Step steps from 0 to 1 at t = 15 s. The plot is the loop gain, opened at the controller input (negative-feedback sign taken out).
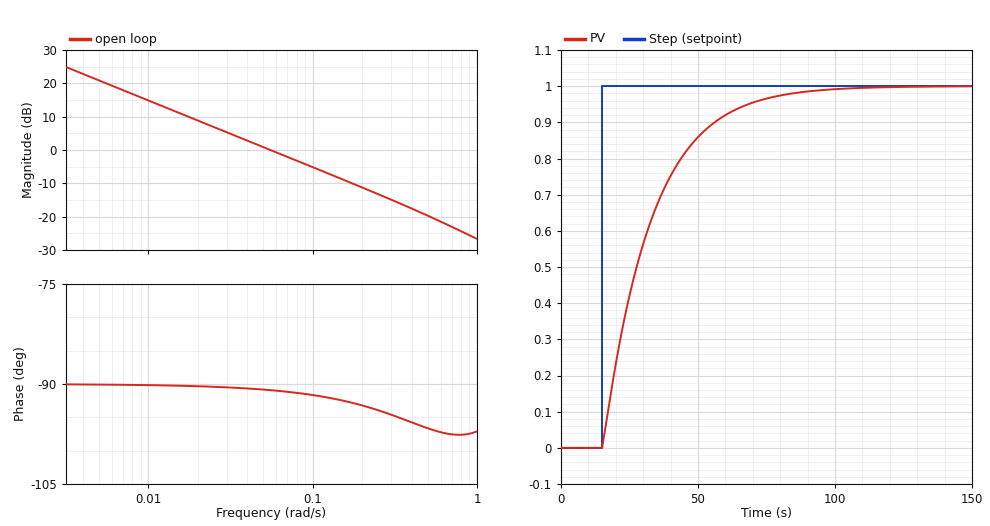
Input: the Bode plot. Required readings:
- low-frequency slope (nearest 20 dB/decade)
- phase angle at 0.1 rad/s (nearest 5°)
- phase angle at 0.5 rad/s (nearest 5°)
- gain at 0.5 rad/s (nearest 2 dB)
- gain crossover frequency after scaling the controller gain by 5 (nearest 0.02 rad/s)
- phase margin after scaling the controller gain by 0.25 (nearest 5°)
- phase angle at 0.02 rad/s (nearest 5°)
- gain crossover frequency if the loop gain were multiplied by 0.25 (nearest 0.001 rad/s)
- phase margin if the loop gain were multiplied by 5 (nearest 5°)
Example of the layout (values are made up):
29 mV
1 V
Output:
-20 dB/decade
-90°
-95°
-20 dB
0.28 rad/s
90°
-90°
0.014 rad/s
85°
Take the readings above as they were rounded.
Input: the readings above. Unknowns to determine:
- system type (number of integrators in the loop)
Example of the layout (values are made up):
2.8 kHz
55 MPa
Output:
1
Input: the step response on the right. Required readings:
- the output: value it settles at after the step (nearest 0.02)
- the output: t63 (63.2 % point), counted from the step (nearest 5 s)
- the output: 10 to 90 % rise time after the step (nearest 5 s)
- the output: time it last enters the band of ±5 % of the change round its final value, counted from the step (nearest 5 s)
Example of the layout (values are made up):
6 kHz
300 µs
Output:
1.00
20 s
40 s
55 s
